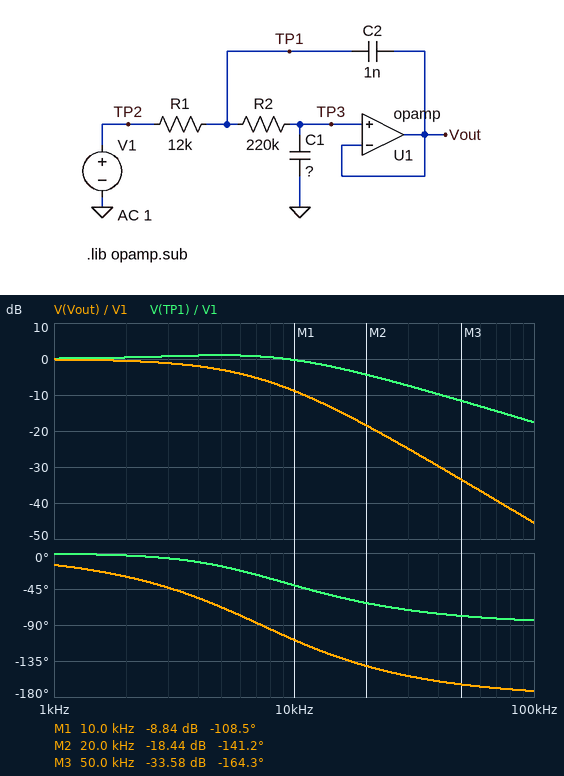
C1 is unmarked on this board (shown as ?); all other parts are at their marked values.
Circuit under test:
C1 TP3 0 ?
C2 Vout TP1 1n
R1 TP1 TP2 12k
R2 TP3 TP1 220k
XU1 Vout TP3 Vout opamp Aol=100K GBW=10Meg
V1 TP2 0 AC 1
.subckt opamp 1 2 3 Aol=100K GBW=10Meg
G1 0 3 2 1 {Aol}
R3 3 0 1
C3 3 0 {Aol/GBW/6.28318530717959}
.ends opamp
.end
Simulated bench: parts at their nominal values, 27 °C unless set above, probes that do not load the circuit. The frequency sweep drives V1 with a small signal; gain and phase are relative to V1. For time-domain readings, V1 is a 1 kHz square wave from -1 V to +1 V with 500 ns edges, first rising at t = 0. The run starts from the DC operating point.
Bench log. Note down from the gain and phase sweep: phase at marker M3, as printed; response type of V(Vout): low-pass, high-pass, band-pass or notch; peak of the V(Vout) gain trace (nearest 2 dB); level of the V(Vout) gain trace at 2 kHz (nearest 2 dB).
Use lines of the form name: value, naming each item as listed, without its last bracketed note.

phase at marker M3, as printed: -164.3 deg
response type of V(Vout): low-pass, high-pass, band-pass or notch: low-pass
peak of the V(Vout) gain trace: 0 dB
level of the V(Vout) gain trace at 2 kHz: 0 dB
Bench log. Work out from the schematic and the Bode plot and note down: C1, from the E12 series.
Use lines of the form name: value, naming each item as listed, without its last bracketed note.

C1, from the E12 series: 180 pF
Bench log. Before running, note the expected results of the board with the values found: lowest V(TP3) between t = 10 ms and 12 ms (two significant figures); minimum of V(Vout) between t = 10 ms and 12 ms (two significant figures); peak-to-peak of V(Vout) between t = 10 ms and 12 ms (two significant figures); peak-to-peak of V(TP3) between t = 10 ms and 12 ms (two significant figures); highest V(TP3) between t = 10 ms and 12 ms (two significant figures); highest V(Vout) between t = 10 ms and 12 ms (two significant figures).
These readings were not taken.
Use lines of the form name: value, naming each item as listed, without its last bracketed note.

lowest V(TP3) between t = 10 ms and 12 ms: -1.0 V
minimum of V(Vout) between t = 10 ms and 12 ms: -1.0 V
peak-to-peak of V(Vout) between t = 10 ms and 12 ms: 2.0 V
peak-to-peak of V(TP3) between t = 10 ms and 12 ms: 2.0 V
highest V(TP3) between t = 10 ms and 12 ms: 1.0 V
highest V(Vout) between t = 10 ms and 12 ms: 1.0 V
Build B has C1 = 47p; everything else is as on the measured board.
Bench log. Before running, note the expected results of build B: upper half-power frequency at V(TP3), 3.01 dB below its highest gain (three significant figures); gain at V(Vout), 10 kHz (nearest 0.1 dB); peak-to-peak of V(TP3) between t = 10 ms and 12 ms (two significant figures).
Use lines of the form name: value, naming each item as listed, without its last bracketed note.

upper half-power frequency at V(TP3), 3.01 dB below its highest gain: 16.7 kHz
gain at V(Vout), 10 kHz: 1.4 dB
peak-to-peak of V(TP3) between t = 10 ms and 12 ms: 2.7 V
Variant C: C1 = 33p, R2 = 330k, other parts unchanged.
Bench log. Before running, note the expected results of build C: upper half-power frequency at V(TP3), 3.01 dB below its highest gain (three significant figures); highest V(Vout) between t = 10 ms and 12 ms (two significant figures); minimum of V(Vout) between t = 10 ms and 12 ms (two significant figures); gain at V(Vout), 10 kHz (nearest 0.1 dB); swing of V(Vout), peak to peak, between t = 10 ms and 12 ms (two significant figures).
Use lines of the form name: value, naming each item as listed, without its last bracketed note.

upper half-power frequency at V(TP3), 3.01 dB below its highest gain: 16.3 kHz
highest V(Vout) between t = 10 ms and 12 ms: 1.3 V
minimum of V(Vout) between t = 10 ms and 12 ms: -1.3 V
gain at V(Vout), 10 kHz: 1.3 dB
swing of V(Vout), peak to peak, between t = 10 ms and 12 ms: 2.7 V
